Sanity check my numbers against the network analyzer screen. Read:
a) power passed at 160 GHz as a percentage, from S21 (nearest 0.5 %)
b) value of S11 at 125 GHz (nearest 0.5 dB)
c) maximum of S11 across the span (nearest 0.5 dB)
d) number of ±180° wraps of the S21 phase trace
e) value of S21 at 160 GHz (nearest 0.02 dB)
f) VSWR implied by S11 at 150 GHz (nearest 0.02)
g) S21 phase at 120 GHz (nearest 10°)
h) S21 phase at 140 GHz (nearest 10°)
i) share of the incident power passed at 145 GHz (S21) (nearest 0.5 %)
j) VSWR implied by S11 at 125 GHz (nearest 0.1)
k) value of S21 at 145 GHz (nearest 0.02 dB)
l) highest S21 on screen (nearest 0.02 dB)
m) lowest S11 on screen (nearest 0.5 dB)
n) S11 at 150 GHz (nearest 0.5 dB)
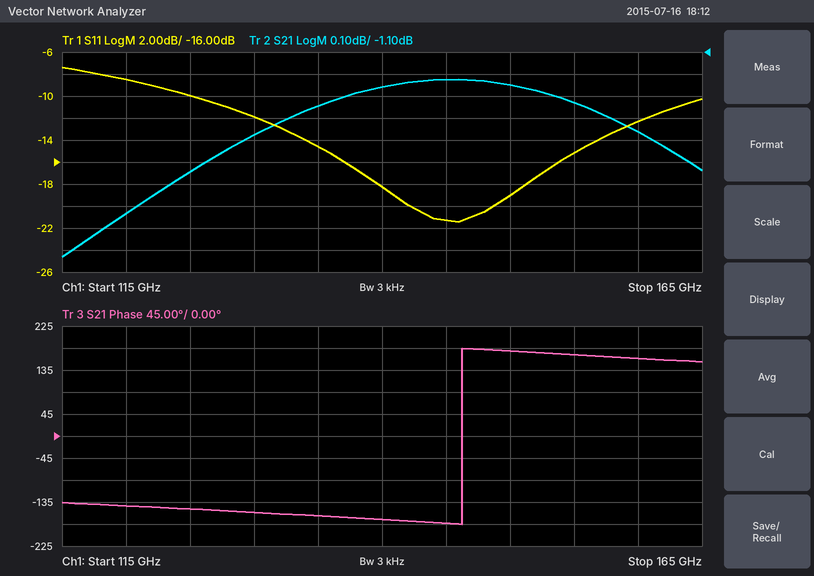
71.5 %
-10.0 dB
-7.5 dB
1
-1.46 dB
1.26
-140°
-170°
75.5 %
1.9
-1.22 dB
-1.22 dB
-21.5 dB
-19.0 dB
